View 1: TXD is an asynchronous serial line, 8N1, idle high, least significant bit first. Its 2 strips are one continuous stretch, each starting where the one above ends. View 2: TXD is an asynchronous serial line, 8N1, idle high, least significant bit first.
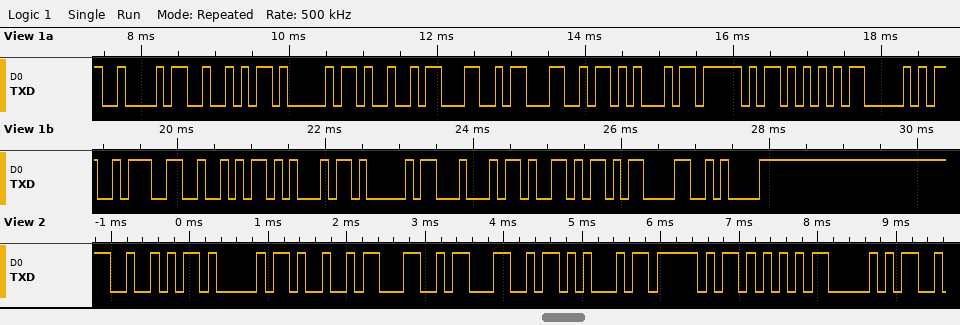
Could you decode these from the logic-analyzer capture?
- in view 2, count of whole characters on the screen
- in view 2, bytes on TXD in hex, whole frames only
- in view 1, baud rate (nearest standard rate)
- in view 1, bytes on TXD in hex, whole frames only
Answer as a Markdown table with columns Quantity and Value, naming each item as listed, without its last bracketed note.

| Quantity | Value |
|---|---|
| in view 2, count of whole characters on the screen | 9 |
| in view 2, bytes on TXD in hex, whole frames only | 52 41 49 4C 4C 45 5F 55 50 |
| in view 1, baud rate | 9600 baud |
| in view 1, bytes on TXD in hex, whole frames only | 42 52 41 49 4C 4C 45 5F 55 50 3A 52 45 41 44 59 0D 0A |
